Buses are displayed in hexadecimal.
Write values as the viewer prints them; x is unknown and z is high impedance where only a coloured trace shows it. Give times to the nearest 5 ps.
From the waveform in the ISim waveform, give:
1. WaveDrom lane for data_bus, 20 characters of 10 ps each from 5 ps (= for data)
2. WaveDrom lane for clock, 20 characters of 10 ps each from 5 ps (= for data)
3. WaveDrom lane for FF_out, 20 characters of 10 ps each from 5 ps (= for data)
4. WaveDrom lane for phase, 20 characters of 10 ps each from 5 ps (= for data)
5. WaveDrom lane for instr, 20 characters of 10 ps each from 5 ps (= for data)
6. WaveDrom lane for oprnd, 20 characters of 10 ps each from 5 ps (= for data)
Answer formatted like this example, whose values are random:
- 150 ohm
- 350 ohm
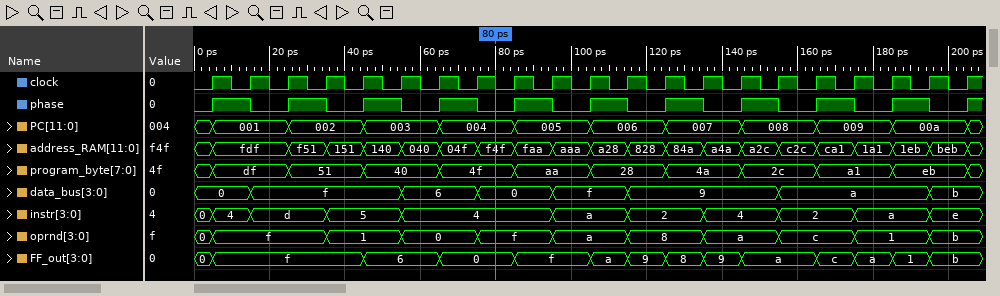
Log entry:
- {name: 'data_bus', wave: '==...=.=.=.=...=...=', data: '0 f 6 0 f 9 a b'}
- {name: 'clock', wave: 'p...................'}
- {name: 'FF_out', wave: '=...=.=.=.=====.====', data: 'f 6 0 f a 9 8 9 a c a 1 b'}
- {name: 'phase', wave: '10101010101010101010'}
- {name: 'instr', wave: '==.=.=...=.=.=.=.=.=', data: '4 d 5 4 a 2 4 2 a e'}
- {name: 'oprnd', wave: '=..=.=.=.=.=.=.=.=.=', data: 'f 1 0 f a 8 a c 1 b'}
